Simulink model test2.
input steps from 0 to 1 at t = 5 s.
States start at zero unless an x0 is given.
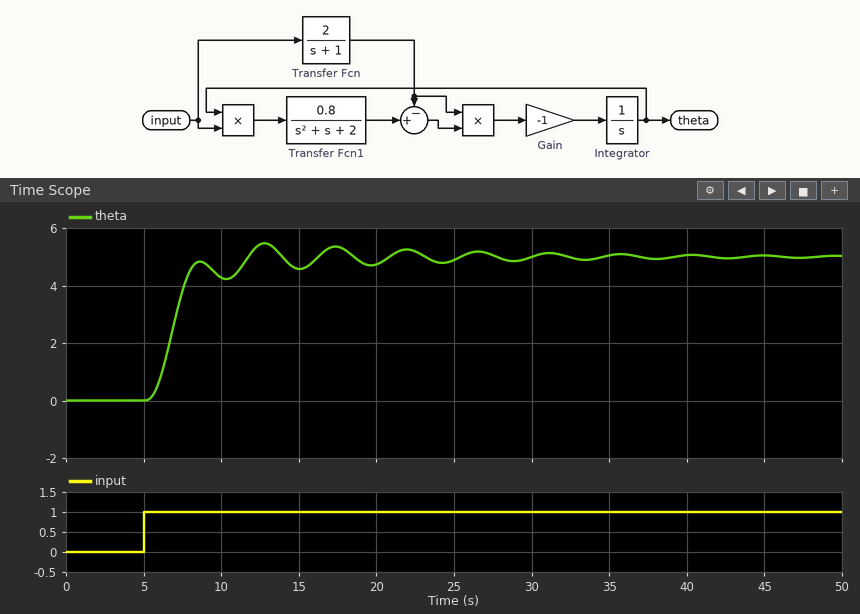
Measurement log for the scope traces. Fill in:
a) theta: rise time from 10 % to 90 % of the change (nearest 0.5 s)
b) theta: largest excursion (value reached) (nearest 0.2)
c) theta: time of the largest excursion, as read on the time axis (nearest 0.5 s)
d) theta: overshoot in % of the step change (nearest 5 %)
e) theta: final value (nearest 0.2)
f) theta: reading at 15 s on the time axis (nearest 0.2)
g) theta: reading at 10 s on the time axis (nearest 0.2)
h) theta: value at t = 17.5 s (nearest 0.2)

2.0 s
5.4
13.0 s
10 %
5.0
4.6
4.2
5.4
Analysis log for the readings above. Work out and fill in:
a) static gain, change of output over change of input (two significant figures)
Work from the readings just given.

5.0
